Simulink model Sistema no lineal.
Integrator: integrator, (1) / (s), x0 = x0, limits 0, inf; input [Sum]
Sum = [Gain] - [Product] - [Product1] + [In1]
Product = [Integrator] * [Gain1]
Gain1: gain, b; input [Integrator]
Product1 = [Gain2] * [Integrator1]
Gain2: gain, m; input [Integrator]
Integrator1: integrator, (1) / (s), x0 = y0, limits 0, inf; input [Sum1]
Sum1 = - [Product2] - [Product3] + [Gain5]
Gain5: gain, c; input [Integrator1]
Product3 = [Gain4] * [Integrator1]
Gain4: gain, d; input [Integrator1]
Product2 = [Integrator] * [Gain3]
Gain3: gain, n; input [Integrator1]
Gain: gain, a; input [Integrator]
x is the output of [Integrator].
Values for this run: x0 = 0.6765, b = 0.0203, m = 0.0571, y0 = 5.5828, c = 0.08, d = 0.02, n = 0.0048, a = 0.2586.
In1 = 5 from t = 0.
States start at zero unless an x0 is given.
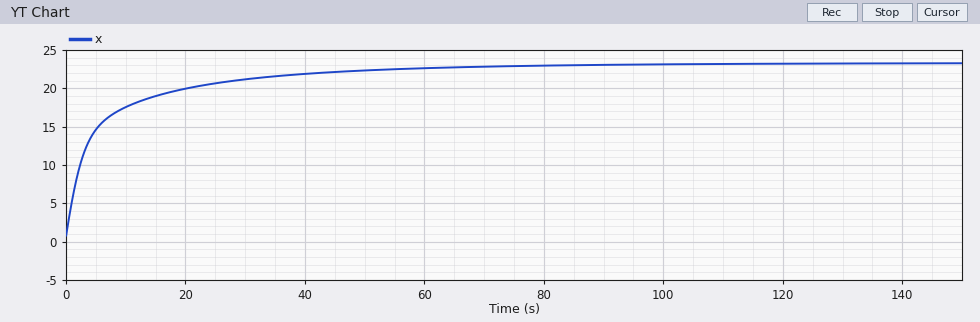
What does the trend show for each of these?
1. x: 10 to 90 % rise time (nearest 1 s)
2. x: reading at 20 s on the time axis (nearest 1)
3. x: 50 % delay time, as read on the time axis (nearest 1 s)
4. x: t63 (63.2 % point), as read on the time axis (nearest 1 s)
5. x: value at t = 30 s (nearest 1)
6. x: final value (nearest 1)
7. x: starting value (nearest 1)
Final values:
28 s
20
3 s
5 s
21
23
1
